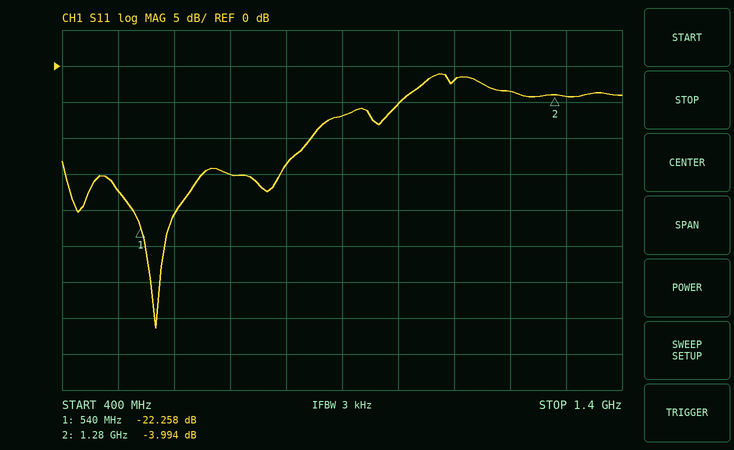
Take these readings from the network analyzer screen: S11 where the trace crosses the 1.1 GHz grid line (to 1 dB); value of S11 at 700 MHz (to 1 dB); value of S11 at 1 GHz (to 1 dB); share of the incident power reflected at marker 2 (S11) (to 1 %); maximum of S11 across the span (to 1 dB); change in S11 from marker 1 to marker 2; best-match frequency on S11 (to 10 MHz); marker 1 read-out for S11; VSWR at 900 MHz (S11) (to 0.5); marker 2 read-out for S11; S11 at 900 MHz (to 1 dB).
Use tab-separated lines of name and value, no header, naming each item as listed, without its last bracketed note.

S11 where the trace crosses the 1.1 GHz grid line	-2 dB
value of S11 at 700 MHz	-15 dB
value of S11 at 1 GHz	-5 dB
share of the incident power reflected at marker 2 (S11)	40 %
maximum of S11 across the span	-1 dB
change in S11 from marker 1 to marker 2	18.264 dB
best-match frequency on S11	570 MHz
marker 1 read-out for S11	-22.258 dB
VSWR at 900 MHz (S11)	2.5
marker 2 read-out for S11	-3.994 dB
S11 at 900 MHz	-7 dB
